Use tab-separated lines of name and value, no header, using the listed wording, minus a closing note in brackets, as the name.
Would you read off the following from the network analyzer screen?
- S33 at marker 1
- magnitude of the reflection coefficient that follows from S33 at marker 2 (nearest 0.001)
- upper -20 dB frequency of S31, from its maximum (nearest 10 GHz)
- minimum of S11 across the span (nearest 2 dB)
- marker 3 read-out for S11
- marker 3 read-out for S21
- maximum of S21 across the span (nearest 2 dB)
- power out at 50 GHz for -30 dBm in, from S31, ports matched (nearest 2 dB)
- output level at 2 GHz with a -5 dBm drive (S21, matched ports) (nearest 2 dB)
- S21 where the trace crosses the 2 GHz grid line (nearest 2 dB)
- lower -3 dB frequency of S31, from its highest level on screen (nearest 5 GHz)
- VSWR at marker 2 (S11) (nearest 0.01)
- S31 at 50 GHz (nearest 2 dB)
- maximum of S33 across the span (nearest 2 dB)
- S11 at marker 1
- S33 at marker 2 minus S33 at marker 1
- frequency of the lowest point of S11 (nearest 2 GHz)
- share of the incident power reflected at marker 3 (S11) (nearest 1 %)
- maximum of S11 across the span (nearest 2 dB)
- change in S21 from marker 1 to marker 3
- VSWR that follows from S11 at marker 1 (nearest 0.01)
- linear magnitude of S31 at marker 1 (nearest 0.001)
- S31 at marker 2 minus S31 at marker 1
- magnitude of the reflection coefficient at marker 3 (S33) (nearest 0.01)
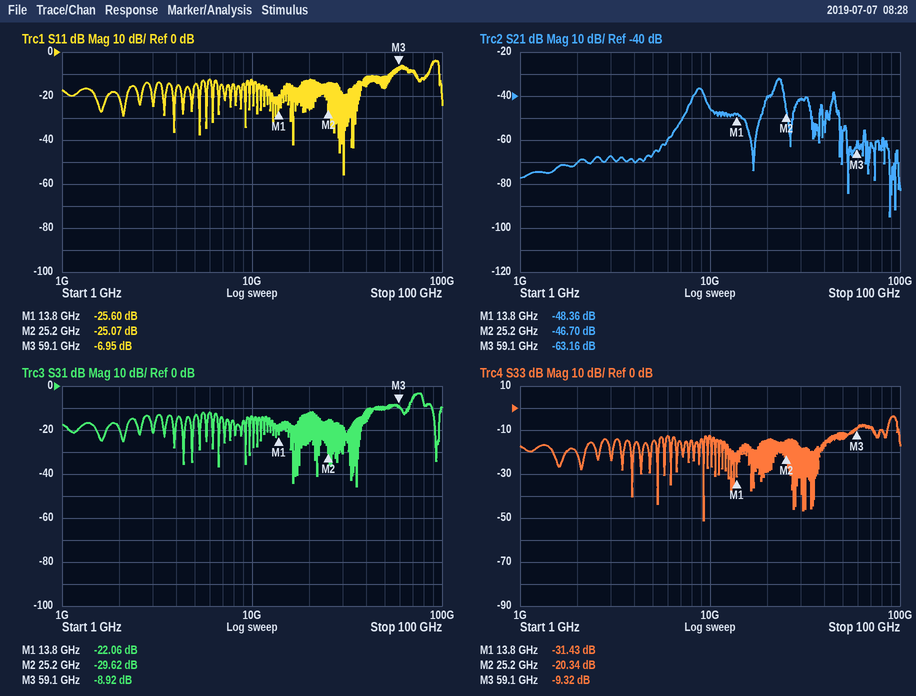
S33 at marker 1	-31.43 dB
magnitude of the reflection coefficient that follows from S33 at marker 2	0.096
upper -20 dB frequency of S31, from its maximum	90 GHz
minimum of S11 across the span	-56 dB
marker 3 read-out for S11	-6.95 dB
marker 3 read-out for S21	-63.16 dB
maximum of S21 across the span	-32 dB
power out at 50 GHz for -30 dBm in, from S31, ports matched	-40 dBm
output level at 2 GHz with a -5 dBm drive (S21, matched ports)	-76 dBm
S21 where the trace crosses the 2 GHz grid line	-70 dB
lower -3 dB frequency of S31, from its highest level on screen	70 GHz
VSWR at marker 2 (S11)	1.12
S31 at 50 GHz	-10 dB
maximum of S33 across the span	-4 dB
S11 at marker 1	-25.60 dB
S33 at marker 2 minus S33 at marker 1	11.09 dB
frequency of the lowest point of S11	30 GHz
share of the incident power reflected at marker 3 (S11)	20 %
maximum of S11 across the span	-4 dB
change in S21 from marker 1 to marker 3	-14.80 dB
VSWR that follows from S11 at marker 1	1.11
linear magnitude of S31 at marker 1	0.079
S31 at marker 2 minus S31 at marker 1	-7.56 dB
magnitude of the reflection coefficient at marker 3 (S33)	0.34
